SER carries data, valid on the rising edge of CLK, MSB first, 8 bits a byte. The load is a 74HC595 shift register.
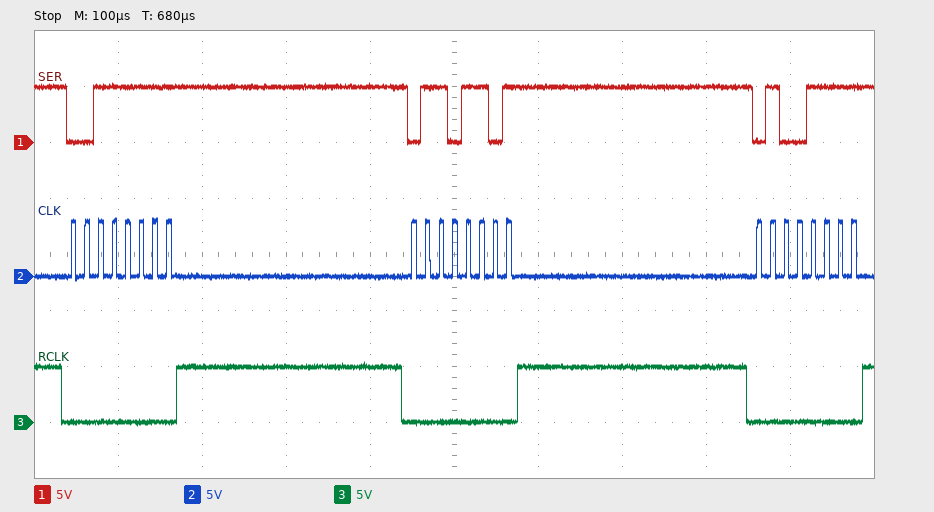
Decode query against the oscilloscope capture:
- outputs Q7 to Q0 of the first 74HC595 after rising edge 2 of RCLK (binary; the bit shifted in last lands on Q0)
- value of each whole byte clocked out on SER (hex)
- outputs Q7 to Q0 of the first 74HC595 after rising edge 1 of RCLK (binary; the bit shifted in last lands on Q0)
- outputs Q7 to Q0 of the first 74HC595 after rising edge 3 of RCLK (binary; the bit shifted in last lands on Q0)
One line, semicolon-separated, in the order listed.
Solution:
01101101; 3F 6D 4F; 00111111; 01001111
